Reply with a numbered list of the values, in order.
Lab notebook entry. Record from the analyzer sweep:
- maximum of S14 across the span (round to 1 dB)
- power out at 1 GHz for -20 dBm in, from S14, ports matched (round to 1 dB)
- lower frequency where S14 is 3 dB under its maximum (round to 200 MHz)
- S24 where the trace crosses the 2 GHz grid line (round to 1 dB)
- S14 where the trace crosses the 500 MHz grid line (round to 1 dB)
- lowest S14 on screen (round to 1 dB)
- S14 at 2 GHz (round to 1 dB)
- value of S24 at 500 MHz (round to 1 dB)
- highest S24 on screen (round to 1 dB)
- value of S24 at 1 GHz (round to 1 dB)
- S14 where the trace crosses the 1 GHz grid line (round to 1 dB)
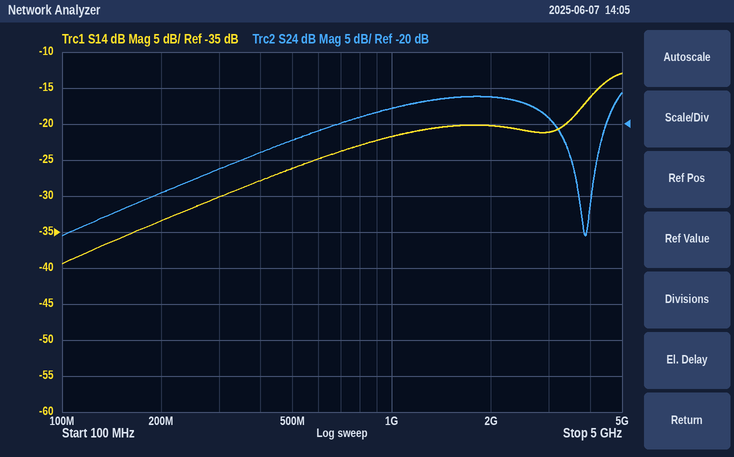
1. -13 dB
2. -42 dBm
3. 4.0 GHz
4. -16 dB
5. -26 dB
6. -39 dB
7. -20 dB
8. -22 dB
9. -16 dB
10. -18 dB
11. -22 dB
